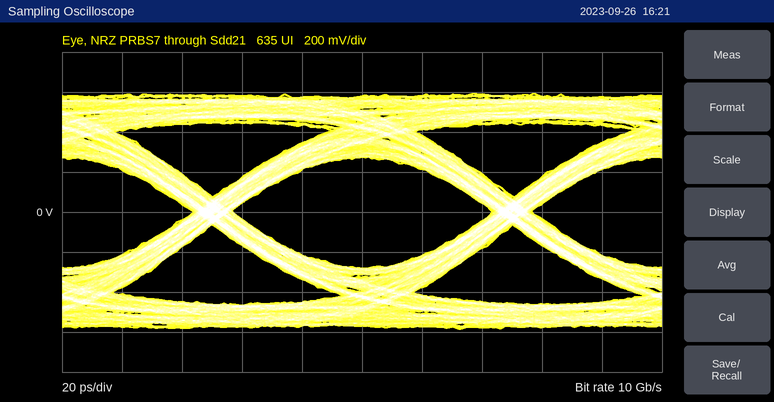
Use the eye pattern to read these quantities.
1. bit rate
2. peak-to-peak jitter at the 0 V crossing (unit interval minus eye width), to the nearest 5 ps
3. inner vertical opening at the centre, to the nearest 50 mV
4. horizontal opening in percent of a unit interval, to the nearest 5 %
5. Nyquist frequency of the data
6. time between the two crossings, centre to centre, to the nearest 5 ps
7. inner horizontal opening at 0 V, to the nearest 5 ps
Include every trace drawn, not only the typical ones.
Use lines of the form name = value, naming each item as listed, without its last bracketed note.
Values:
bit rate = 10 Gb/s
peak-to-peak jitter at the 0 V crossing (unit interval minus eye width), to the nearest 5 ps = 15 ps
inner vertical opening at the centre, to the nearest 50 mV = 550 mV
horizontal opening in percent of a unit interval, to the nearest 5 % = 85 %
Nyquist frequency of the data = 5 GHz
time between the two crossings, centre to centre, to the nearest 5 ps = 100 ps
inner horizontal opening at 0 V, to the nearest 5 ps = 85 ps
